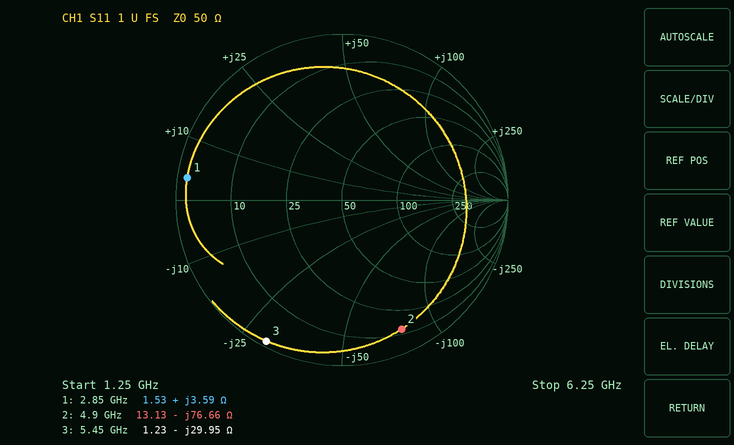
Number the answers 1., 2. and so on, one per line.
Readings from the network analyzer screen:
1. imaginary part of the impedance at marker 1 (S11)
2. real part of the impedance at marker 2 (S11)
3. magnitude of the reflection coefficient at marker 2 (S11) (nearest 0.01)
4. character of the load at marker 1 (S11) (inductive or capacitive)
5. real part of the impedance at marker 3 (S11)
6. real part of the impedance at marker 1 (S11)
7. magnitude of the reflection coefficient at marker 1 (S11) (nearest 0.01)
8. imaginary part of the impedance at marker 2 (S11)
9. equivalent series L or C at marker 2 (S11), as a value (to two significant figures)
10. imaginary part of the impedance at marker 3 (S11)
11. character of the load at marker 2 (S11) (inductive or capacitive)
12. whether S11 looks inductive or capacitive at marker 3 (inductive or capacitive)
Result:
1. +3.59 Ω
2. 13.13 Ω
3. 0.86
4. inductive
5. 1.23 Ω
6. 1.53 Ω
7. 0.94
8. -76.66 Ω
9. 420 fF
10. -29.95 Ω
11. capacitive
12. capacitive
